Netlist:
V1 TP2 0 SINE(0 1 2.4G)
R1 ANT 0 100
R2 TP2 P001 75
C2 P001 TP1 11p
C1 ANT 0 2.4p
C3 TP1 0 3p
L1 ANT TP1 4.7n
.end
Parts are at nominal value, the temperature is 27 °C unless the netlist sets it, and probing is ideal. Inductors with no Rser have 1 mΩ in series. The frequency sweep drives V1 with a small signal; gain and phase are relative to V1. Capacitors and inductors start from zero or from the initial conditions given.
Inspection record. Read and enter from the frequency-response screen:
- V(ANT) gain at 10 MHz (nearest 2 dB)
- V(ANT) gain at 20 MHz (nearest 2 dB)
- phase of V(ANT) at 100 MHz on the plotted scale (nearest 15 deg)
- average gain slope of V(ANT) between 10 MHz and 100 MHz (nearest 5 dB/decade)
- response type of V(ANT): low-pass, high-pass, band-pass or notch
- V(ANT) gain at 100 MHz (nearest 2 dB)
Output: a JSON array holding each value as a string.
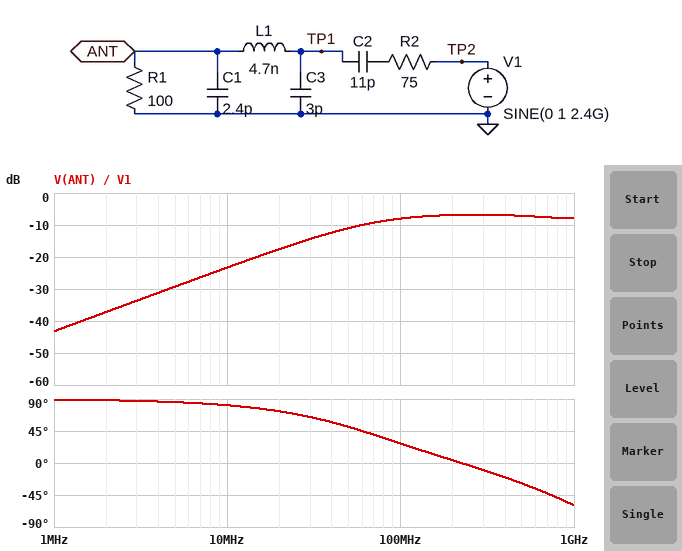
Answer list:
["-24 dB", "-18 dB", "30 deg", "15 dB/decade", "high-pass", "-8 dB"]
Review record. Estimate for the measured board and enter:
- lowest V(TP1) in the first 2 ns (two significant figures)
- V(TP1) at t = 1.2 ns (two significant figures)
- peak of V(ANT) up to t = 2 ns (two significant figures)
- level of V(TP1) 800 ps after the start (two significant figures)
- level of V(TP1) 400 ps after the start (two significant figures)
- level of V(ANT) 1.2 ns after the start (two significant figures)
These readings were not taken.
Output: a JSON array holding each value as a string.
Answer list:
["-480 mV", "-480 mV", "310 mV", "-460 mV", "-280 mV", "270 mV"]
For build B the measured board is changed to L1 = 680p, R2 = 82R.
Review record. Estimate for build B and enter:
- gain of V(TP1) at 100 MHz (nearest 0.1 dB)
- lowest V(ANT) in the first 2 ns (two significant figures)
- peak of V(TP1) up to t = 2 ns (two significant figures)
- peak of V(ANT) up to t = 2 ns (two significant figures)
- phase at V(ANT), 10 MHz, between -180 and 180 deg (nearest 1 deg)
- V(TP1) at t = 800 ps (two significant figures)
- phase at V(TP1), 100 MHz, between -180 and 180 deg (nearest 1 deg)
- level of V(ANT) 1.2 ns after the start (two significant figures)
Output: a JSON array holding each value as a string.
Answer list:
["-8.3 dB", "-190 mV", "160 mV", "250 mV", "81 deg", "-120 mV", "27 deg", "-170 mV"]
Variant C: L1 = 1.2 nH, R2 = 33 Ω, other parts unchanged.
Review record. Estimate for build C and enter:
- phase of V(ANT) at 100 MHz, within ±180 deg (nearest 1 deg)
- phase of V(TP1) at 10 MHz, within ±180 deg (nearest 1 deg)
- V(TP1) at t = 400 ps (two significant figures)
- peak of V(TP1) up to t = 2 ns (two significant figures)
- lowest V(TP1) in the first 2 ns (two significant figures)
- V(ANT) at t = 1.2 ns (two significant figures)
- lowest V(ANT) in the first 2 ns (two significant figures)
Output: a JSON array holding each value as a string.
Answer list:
["36 deg", "83 deg", "-130 mV", "360 mV", "-220 mV", "-470 mV", "-570 mV"]
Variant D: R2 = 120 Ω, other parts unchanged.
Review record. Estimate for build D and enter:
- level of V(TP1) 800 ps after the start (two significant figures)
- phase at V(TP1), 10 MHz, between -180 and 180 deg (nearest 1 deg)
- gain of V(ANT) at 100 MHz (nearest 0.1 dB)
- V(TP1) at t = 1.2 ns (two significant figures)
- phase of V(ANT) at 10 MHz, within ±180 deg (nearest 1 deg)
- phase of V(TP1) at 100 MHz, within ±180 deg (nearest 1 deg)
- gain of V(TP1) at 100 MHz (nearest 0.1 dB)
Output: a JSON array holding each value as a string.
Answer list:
["-340 mV", "80 deg", "-9.1 dB", "-330 mV", "79 deg", "22 deg", "-9.2 dB"]
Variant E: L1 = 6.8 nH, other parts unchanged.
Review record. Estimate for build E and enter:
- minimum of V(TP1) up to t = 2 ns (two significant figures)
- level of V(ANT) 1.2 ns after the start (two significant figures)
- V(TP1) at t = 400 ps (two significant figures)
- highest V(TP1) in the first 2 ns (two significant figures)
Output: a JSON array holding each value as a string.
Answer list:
["-410 mV", "95 mV", "-340 mV", "420 mV"]
